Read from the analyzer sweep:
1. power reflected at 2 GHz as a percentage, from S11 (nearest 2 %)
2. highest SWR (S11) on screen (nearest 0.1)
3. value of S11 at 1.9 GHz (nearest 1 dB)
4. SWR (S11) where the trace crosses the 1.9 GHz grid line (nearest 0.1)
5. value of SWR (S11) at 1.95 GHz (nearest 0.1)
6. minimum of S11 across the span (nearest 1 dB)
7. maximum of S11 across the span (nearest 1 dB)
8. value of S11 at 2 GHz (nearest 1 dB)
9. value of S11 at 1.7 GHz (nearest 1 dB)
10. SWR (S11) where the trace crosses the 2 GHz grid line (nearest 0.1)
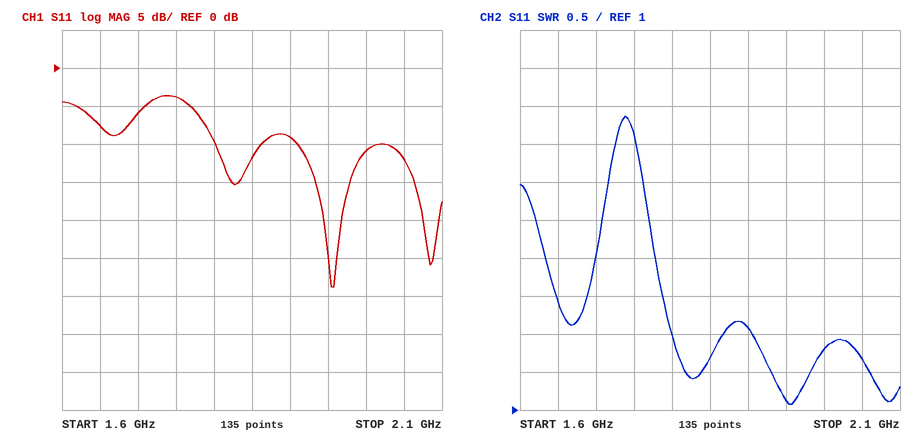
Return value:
8 %
4.9
-9 dB
2.1
1.1
-29 dB
-4 dB
-11 dB
-6 dB
1.8
